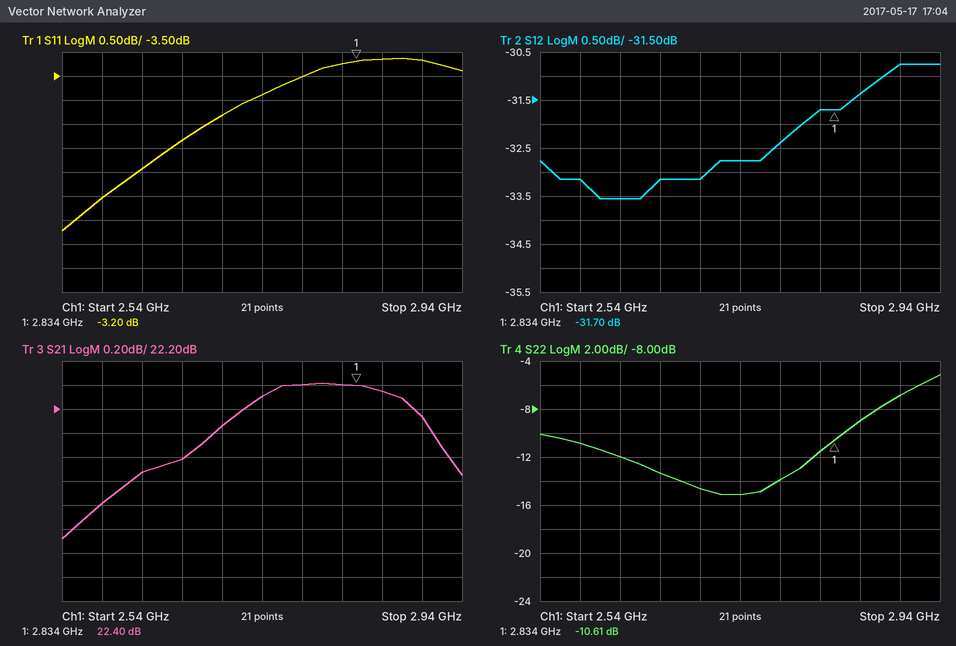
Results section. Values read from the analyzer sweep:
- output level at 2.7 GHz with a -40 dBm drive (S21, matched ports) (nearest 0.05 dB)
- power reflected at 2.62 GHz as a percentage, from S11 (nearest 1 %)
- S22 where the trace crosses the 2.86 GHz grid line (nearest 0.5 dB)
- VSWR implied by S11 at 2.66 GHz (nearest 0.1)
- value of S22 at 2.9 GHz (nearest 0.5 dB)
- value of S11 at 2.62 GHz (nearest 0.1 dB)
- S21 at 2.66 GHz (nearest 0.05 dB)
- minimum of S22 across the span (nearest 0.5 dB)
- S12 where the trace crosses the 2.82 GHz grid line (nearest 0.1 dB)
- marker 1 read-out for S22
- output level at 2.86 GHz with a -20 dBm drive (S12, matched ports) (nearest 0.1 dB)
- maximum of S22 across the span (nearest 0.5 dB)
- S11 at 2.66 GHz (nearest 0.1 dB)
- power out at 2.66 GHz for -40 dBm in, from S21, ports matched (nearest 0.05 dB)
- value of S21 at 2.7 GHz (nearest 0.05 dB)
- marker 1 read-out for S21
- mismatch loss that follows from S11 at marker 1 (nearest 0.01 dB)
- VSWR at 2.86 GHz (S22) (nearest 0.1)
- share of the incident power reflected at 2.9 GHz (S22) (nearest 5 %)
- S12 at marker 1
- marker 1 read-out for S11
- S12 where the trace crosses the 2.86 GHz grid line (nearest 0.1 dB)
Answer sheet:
-17.95 dBm
29 %
-9.0 dB
3.7
-7.0 dB
-5.4 dB
21.80 dB
-15.0 dB
-31.7 dB
-10.61 dB
-51.4 dBm
-5.0 dB
-4.8 dB
-18.20 dBm
22.05 dB
22.40 dB
2.83 dB
2.1
20 %
-31.70 dB
-3.20 dB
-31.4 dB
